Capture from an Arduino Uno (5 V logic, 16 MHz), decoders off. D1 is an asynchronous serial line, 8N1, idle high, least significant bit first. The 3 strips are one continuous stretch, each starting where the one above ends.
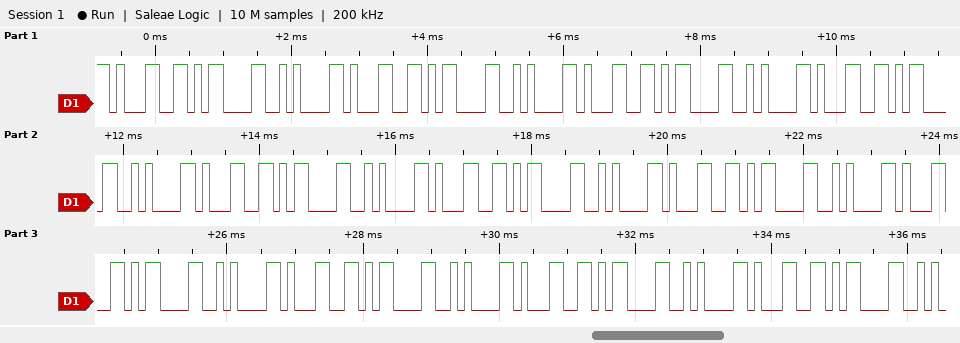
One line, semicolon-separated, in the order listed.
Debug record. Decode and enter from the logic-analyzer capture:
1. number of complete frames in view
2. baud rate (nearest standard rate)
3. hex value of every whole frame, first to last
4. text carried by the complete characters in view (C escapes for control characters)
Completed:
32; 9600 baud; 0x31 0x0D 0x0A 0x31 0x0D 0x0A 0x31 0x0D 0x0A 0x31 0x0D 0x0A 0x31 0x0D 0x0A 0x31 0x0D 0x0A 0x31 0x0D 0x0A 0x31 0x0D 0x0A 0x31 0x0D 0x0A 0x31 0x0D 0x0A 0x31 0x0D; "1\r\n1\r\n1\r\n1\r\n1\r\n1\r\n1\r\n1\r\n1\r\n1\r\n1\r"
